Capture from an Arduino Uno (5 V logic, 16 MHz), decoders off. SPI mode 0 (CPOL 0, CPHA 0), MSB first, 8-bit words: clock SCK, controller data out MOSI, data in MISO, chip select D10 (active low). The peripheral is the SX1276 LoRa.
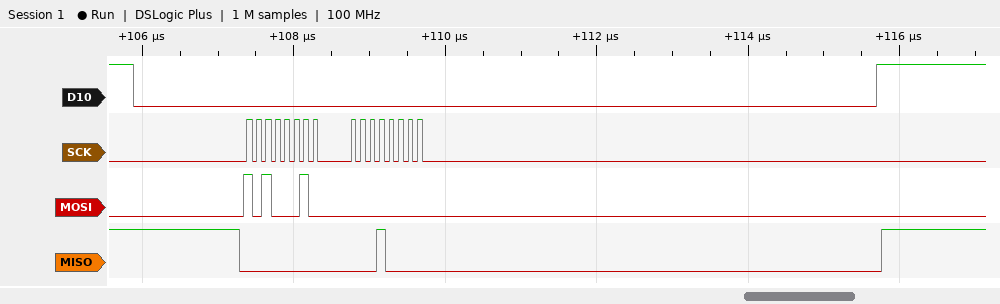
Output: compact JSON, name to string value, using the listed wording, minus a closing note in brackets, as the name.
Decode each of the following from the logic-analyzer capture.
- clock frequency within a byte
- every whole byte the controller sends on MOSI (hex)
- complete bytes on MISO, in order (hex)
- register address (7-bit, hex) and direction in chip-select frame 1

{"clock frequency within a byte": "8 MHz", "every whole byte the controller sends on MOSI": "A2 00", "complete bytes on MISO, in order": "00 10", "register address (7-bit, hex) and direction in chip-select frame 1": "0x22 write"}
